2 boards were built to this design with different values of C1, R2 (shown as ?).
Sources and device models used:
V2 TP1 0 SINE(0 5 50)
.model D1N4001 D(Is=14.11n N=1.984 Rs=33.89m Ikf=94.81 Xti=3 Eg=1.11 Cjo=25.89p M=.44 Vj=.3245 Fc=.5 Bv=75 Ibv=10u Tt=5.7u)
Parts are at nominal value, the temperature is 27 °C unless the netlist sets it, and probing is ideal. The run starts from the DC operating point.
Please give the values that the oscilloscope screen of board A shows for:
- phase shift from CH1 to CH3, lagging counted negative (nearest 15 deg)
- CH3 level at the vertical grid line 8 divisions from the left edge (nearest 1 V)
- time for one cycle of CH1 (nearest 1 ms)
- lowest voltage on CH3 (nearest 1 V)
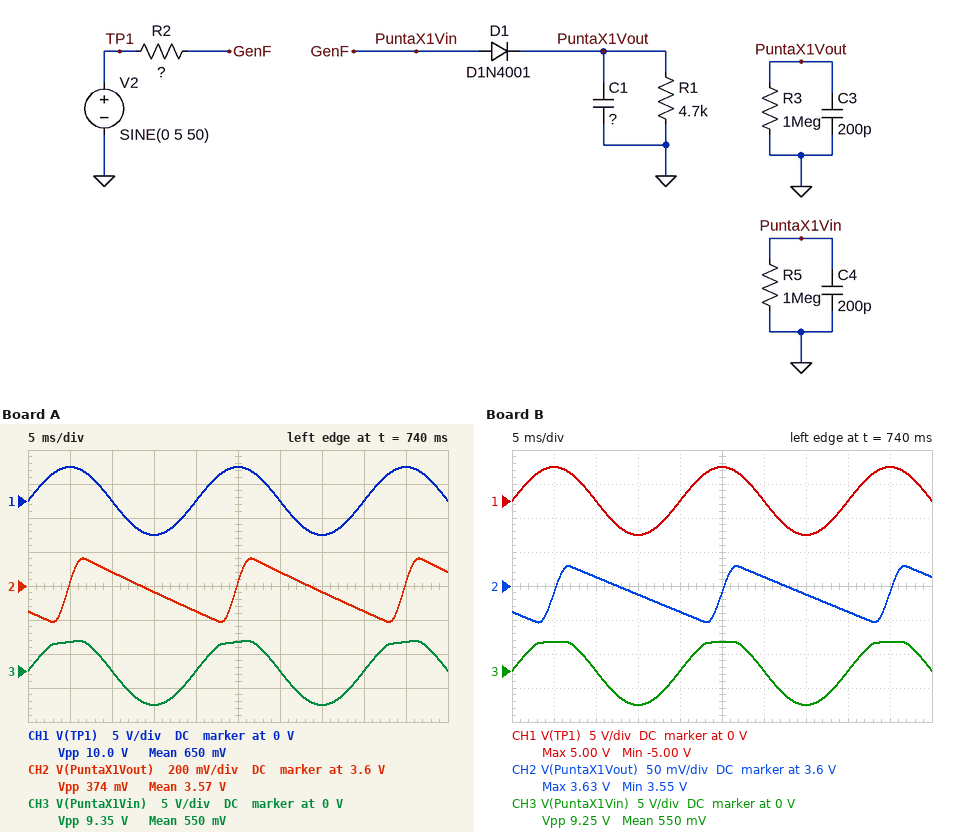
0 deg
0 V
20 ms
-5 V
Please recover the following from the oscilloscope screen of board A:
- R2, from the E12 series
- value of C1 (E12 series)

120 Ω
33 µF
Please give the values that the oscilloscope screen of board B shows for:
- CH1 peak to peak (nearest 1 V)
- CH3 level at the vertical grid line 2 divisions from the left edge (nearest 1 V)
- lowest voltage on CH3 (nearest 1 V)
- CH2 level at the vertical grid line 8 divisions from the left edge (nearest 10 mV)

10 V
0 V
-5 V
3.56 V
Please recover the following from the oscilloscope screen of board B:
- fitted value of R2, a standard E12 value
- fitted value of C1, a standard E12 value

120 Ω
150 µF
